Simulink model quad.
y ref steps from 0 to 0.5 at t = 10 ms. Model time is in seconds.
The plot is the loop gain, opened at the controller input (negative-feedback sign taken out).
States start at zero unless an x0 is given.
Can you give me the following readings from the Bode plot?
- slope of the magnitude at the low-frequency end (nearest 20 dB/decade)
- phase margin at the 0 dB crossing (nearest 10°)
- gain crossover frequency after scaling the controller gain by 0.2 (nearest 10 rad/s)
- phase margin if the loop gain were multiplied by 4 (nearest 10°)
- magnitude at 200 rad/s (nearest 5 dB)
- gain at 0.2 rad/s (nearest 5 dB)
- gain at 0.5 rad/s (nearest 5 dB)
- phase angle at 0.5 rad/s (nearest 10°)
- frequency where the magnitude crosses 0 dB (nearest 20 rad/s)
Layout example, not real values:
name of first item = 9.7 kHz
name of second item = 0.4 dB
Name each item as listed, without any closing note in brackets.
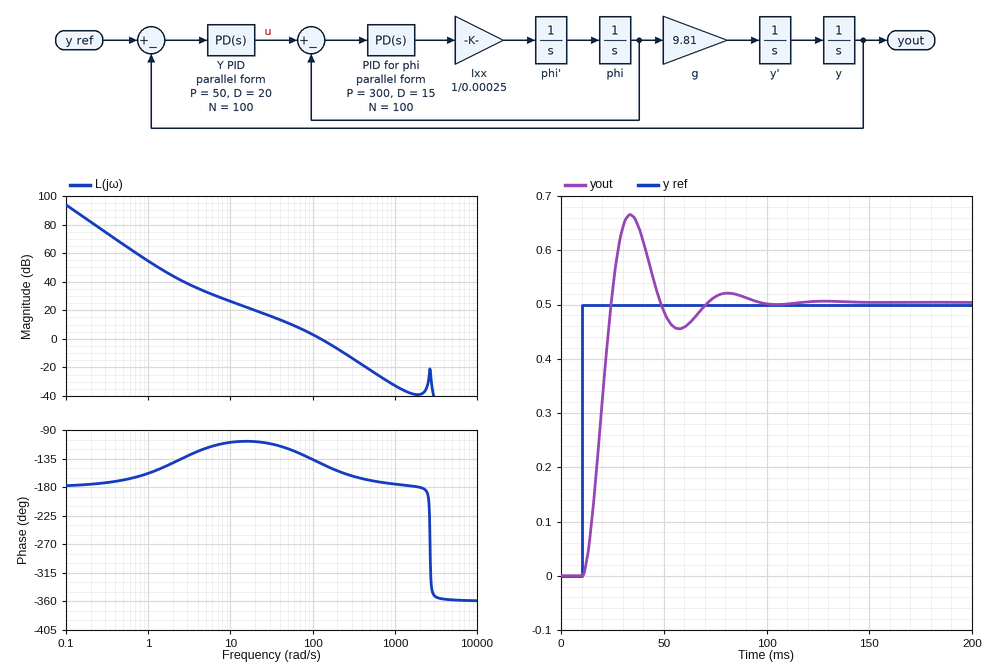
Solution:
slope of the magnitude at the low-frequency end = -40 dB/decade
phase margin at the 0 dB crossing = 40°
gain crossover frequency after scaling the controller gain by 0.2 = 40 rad/s
phase margin if the loop gain were multiplied by 4 = 20°
magnitude at 200 rad/s = -5 dB
gain at 0.2 rad/s = 80 dB
gain at 0.5 rad/s = 65 dB
phase angle at 0.5 rad/s = -170°
frequency where the magnitude crosses 0 dB = 120 rad/s
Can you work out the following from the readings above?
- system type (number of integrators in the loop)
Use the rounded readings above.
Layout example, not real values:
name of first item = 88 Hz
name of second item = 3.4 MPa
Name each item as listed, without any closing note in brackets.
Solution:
system type = 2
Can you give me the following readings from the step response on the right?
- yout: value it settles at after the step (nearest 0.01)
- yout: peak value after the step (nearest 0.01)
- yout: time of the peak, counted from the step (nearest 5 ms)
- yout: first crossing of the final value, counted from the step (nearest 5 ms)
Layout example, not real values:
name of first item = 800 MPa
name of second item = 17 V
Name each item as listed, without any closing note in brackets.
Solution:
yout: value it settles at after the step = 0.50
yout: peak value after the step = 0.67
yout: time of the peak, counted from the step = 25 ms
yout: first crossing of the final value, counted from the step = 15 ms
